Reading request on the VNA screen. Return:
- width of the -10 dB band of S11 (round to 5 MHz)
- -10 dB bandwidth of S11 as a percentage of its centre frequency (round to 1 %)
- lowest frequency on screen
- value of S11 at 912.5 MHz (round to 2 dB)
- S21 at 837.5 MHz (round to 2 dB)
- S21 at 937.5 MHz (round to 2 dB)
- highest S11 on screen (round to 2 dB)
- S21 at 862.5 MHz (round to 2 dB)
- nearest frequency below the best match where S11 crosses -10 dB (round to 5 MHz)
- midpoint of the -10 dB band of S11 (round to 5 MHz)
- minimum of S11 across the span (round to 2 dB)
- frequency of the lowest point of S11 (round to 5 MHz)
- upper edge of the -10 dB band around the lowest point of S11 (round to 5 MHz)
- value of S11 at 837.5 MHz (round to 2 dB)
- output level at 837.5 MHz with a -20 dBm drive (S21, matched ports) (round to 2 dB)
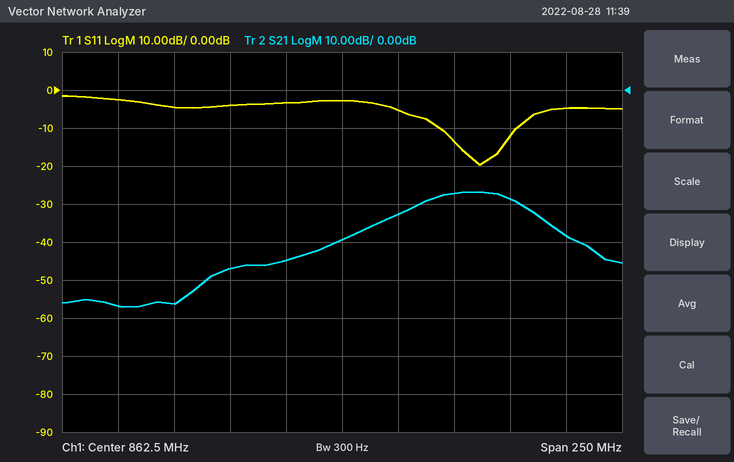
35 MHz
4 %
737.5 MHz
-14 dB
-44 dB
-28 dB
-2 dB
-40 dB
905 MHz
925 MHz
-20 dB
925 MHz
940 MHz
-4 dB
-64 dBm
